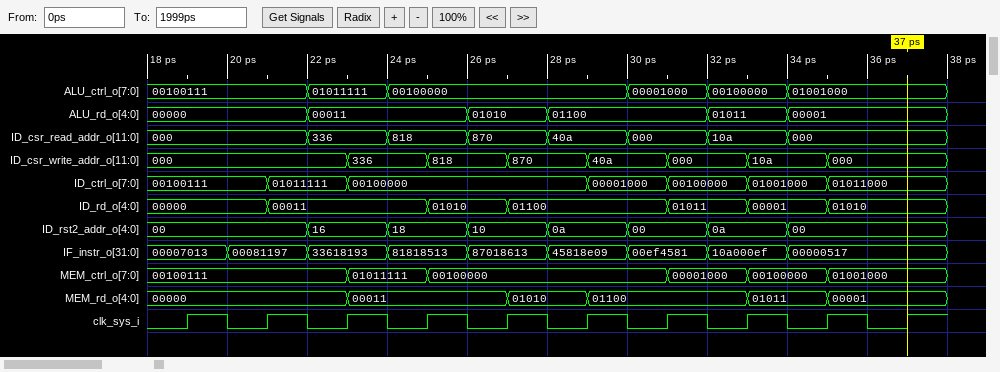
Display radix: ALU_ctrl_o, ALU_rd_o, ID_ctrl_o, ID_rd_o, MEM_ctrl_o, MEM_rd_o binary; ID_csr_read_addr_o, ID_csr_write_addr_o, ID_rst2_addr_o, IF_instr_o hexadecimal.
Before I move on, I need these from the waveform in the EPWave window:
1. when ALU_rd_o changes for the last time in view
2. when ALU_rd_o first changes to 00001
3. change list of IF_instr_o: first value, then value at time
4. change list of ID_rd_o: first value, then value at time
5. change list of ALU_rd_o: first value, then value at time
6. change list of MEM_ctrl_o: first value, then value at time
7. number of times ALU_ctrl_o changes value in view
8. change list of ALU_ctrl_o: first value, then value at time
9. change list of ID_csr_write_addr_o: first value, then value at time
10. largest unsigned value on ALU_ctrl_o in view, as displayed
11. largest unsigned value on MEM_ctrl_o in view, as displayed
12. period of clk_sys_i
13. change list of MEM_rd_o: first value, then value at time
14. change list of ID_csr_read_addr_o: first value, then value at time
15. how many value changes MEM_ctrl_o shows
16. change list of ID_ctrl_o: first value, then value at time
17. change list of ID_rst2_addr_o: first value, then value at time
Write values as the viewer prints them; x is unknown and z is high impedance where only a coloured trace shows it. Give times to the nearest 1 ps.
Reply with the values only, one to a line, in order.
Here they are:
34 ps
34 ps
00007013, 00081197 at 20 ps, 33618193 at 22 ps, 81818513 at 24 ps, 87018613 at 26 ps, 45818e09 at 28 ps, 00ef4581 at 30 ps, 10a000ef at 32 ps, 00000517 at 34 ps
00000, 00011 at 21 ps, 01010 at 25 ps, 01100 at 27 ps, 01011 at 31 ps, 00001 at 33 ps, 01010 at 35 ps
00000, 00011 at 22 ps, 01010 at 26 ps, 01100 at 28 ps, 01011 at 32 ps, 00001 at 34 ps
00100111, 01011111 at 23 ps, 00100000 at 25 ps, 00001000 at 31 ps, 00100000 at 33 ps, 01001000 at 35 ps
5
00100111, 01011111 at 22 ps, 00100000 at 24 ps, 00001000 at 30 ps, 00100000 at 32 ps, 01001000 at 34 ps
000, 336 at 23 ps, 818 at 25 ps, 870 at 27 ps, 40a at 29 ps, 000 at 31 ps, 10a at 33 ps, 000 at 35 ps
01011111
01011111
2 ps
00000, 00011 at 23 ps, 01010 at 27 ps, 01100 at 29 ps, 01011 at 33 ps, 00001 at 35 ps
000, 336 at 22 ps, 818 at 24 ps, 870 at 26 ps, 40a at 28 ps, 000 at 30 ps, 10a at 32 ps, 000 at 34 ps
5
00100111, 01011111 at 21 ps, 00100000 at 23 ps, 00001000 at 29 ps, 00100000 at 31 ps, 01001000 at 33 ps, 01011000 at 35 ps
00, 16 at 22 ps, 18 at 24 ps, 10 at 26 ps, 0a at 28 ps, 00 at 30 ps, 0a at 32 ps, 00 at 34 ps
